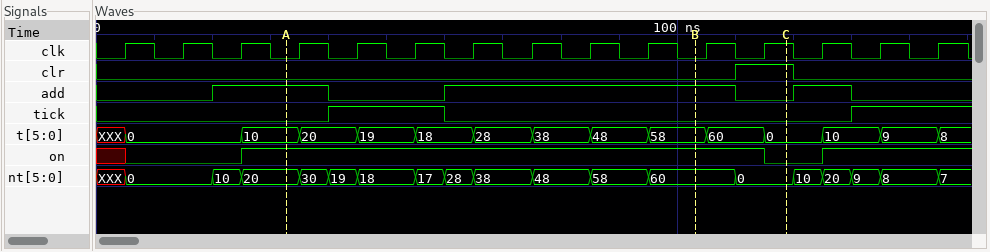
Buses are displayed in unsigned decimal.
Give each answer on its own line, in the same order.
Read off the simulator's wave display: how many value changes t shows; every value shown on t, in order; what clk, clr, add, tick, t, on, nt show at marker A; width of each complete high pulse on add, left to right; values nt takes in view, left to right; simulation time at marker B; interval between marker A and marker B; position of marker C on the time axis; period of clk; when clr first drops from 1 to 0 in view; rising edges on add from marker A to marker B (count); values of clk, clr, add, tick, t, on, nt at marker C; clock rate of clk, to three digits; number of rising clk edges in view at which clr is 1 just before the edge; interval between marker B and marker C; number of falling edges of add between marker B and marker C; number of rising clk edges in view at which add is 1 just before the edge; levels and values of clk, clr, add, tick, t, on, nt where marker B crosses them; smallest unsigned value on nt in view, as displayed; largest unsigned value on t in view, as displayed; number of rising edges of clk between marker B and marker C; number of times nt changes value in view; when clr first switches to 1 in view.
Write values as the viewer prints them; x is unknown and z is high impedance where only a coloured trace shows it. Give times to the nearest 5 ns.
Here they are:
14
XXX, 0, 10, 20, 19, 18, 28, 38, 48, 58, 60, 0, 10, 9, 8
clk=0, clr=0, add=1, tick=0, t=10, on=1, nt=20
20 ns, 50 ns, 10 ns
XXX, 0, 10, 20, 30, 19, 18, 17, 28, 38, 48, 58, 60, 0, 10, 20, 9, 8, 7
105 ns
70 ns
120 ns
10 ns
120 ns
1
clk=1, clr=1, add=0, tick=0, t=0, on=0, nt=0
100 MHz
1
15 ns
1
8
clk=0, clr=0, add=1, tick=0, t=58, on=1, nt=60
0
60
2
18
110 ns
